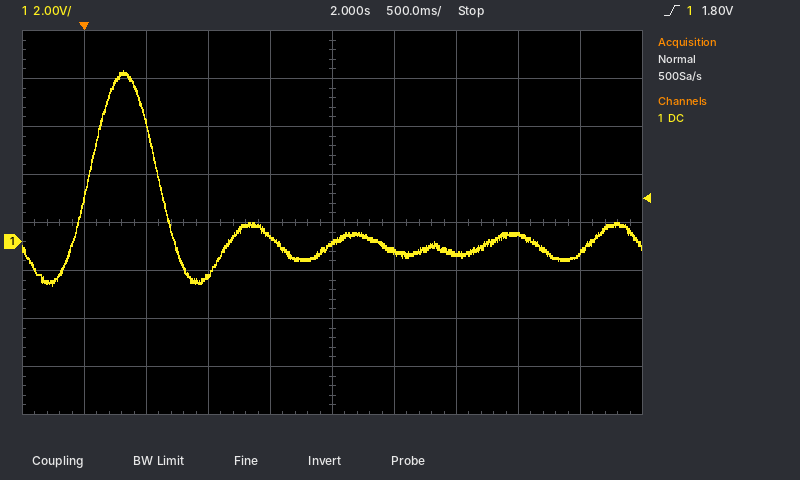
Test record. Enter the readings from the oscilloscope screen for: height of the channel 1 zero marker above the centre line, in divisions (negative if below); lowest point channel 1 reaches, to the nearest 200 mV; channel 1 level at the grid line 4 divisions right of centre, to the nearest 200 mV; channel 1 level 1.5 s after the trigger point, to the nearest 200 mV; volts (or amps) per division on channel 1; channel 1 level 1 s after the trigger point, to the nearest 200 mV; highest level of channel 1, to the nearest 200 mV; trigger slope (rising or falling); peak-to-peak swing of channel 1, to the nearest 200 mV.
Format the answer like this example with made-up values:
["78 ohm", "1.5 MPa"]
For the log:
["-0.4 div", "-1.8 V", "-400 mV", "200 mV", "2 V", "-1.4 V", "7.2 V", "rising", "9.0 V"]
